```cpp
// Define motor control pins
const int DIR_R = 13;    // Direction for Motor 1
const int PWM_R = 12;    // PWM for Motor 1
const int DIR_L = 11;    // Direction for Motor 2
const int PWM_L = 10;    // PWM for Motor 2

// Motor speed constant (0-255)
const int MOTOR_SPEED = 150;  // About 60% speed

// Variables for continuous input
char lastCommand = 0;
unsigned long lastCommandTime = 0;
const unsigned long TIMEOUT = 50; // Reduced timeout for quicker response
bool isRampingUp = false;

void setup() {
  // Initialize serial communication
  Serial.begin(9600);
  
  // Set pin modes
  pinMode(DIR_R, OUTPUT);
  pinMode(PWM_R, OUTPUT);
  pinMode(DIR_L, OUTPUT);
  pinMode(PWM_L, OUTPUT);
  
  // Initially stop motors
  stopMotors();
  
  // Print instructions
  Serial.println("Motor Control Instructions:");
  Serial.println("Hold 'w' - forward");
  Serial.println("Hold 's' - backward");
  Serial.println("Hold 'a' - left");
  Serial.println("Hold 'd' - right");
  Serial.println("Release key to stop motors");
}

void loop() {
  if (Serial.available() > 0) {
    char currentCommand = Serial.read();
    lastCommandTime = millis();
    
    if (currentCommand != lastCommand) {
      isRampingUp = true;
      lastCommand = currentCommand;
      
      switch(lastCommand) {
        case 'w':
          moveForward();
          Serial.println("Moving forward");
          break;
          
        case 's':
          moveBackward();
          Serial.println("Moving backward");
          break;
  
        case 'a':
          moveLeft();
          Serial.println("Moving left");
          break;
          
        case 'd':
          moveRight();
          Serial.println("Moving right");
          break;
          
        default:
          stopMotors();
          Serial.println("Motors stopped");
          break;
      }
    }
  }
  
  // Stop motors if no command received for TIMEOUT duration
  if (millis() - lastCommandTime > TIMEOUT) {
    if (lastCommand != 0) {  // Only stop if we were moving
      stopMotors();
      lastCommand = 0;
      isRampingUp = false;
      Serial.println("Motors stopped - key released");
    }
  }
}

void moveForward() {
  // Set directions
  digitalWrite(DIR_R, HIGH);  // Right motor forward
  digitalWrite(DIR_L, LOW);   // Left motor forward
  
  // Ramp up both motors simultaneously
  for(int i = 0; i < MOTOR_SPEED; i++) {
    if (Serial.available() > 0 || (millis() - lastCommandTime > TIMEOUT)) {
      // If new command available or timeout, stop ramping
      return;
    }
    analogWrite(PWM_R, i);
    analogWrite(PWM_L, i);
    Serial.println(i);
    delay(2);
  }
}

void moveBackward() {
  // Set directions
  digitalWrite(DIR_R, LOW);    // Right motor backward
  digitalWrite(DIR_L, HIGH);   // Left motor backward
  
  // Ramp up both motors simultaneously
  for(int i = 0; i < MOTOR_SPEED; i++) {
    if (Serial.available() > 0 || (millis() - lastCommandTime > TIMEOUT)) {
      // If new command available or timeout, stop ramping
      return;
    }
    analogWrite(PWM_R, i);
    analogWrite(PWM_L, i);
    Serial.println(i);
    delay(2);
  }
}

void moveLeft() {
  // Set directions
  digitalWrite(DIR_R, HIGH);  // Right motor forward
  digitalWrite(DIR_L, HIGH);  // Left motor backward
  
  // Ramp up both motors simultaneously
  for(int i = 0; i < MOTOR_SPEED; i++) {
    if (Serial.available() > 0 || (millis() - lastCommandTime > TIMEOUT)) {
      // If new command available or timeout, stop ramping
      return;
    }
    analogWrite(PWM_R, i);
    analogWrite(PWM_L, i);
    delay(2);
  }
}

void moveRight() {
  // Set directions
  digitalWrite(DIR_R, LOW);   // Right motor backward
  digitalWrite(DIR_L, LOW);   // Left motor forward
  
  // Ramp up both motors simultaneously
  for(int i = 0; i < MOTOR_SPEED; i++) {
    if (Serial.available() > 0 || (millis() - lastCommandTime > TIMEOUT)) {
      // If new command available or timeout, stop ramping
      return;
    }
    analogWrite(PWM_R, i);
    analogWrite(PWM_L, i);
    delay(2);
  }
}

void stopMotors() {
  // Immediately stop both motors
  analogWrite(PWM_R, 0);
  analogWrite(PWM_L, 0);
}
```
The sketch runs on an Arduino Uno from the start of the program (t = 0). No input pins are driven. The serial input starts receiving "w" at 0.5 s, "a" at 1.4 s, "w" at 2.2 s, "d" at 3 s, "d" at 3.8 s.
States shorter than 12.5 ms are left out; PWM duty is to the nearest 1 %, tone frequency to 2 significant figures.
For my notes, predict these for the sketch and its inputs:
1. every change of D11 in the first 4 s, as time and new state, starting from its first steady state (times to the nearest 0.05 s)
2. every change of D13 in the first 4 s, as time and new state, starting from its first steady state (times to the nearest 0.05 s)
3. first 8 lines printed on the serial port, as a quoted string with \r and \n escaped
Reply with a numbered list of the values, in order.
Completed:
1. 0 s low; 1.4 s high; 2.2 s low
2. 0 s low; 0.5 s high; 3 s low
3. "Motor Control Instructions:\r\nHold 'w' - forward\r\nHold 's' - backward\r\nHold 'a' - left\r\nHold 'd' - right\r\nRelease key to stop motors\r\n0\r\n1\r\n"
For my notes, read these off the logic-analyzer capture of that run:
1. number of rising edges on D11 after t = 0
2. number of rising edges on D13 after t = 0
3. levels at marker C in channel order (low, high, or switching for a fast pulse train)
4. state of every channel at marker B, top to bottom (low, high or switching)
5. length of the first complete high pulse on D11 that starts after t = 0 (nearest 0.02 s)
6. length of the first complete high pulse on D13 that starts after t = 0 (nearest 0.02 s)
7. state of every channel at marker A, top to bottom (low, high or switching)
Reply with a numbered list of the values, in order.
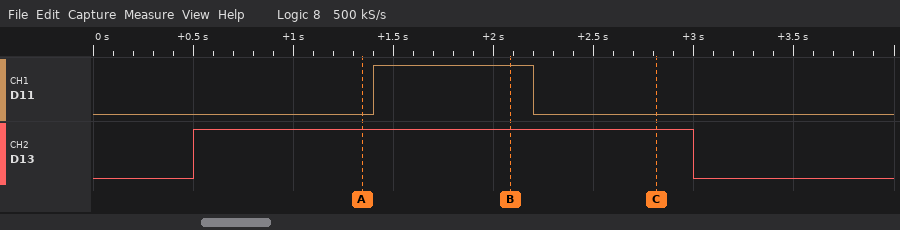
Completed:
1. 1
2. 1
3. D11 low, D13 high
4. D11 high, D13 high
5. 0.80 s
6. 2.50 s
7. D11 low, D13 high
